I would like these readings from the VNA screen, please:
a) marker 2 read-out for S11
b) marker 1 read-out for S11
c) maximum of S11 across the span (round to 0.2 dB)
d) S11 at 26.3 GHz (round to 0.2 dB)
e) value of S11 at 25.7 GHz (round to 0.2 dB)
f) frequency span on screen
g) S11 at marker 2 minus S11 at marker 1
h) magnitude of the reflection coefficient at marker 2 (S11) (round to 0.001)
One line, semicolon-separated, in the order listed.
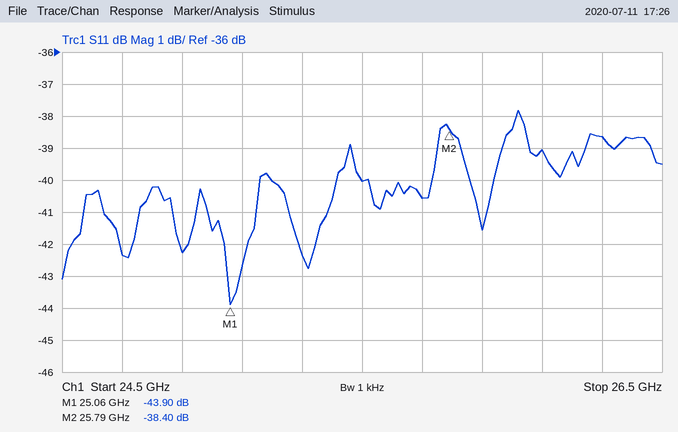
-38.40 dB; -43.90 dB; -37.8 dB; -38.6 dB; -40.6 dB; 2 GHz; 5.50 dB; 0.012
